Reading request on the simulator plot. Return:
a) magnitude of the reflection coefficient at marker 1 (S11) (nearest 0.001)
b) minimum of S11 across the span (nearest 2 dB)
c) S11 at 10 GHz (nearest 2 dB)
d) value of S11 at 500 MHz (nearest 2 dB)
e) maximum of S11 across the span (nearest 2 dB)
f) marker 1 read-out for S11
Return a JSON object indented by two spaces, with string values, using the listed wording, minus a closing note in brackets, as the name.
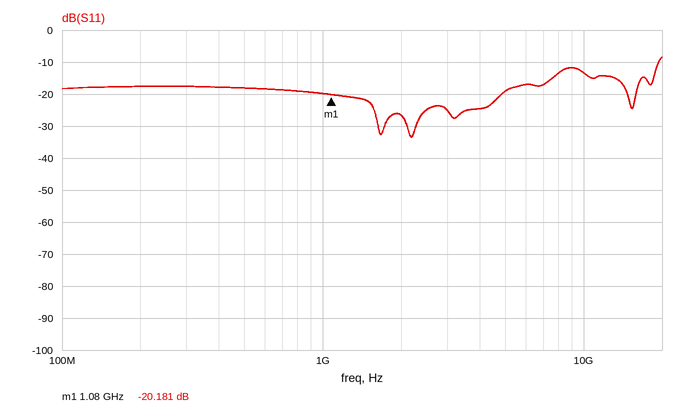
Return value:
{
  "magnitude of the reflection coefficient at marker 1 (S11)": "0.098",
  "minimum of S11 across the span": "-34 dB",
  "S11 at 10 GHz": "-14 dB",
  "value of S11 at 500 MHz": "-18 dB",
  "maximum of S11 across the span": "-8 dB",
  "marker 1 read-out for S11": "-20.181 dB"
}
